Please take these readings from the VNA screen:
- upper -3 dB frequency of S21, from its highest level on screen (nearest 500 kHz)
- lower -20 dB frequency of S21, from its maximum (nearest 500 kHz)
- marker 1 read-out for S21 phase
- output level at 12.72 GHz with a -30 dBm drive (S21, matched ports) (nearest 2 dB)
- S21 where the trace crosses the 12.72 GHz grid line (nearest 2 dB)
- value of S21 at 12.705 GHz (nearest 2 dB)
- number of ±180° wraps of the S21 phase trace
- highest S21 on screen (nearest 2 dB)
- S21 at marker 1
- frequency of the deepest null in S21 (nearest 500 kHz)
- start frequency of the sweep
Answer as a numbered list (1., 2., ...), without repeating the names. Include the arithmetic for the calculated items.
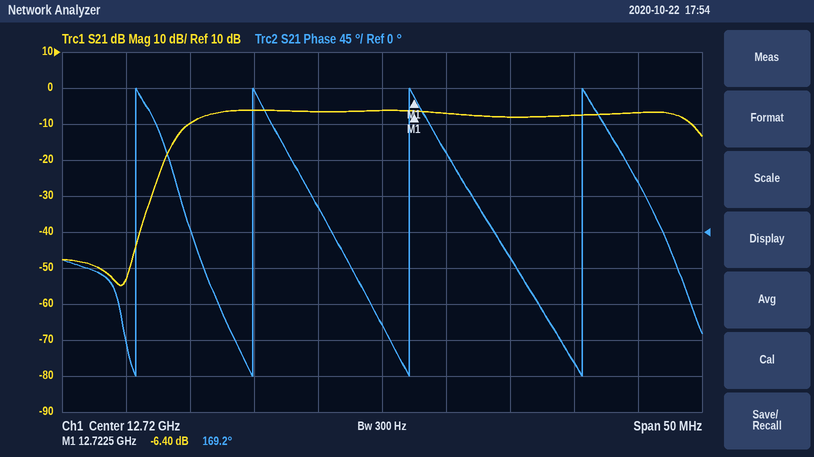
1. 12.7440 GHz
2. 12.7025 GHz
3. 169.2°
4. -30 dBm + (-6 dB) = -36 dBm
5. -6 dB
6. -10 dB
7. 4
8. -6 dB
9. -6.40 dB
10. 12.6995 GHz
11. 12.695 GHz
